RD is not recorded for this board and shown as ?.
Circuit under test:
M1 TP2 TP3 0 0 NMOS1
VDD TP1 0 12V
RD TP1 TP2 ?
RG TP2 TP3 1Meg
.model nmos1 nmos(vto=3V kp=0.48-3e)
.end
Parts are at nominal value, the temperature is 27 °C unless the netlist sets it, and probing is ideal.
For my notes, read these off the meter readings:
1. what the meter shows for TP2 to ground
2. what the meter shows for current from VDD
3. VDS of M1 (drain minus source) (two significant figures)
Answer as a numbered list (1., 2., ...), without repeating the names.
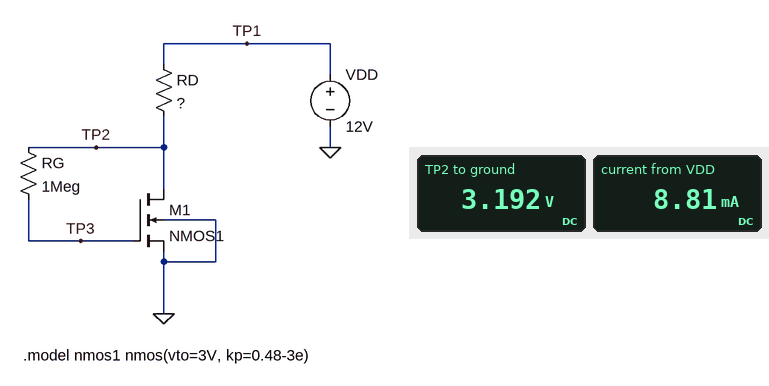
1. 3.192 V
2. 8.81 mA
3. 3.2 V
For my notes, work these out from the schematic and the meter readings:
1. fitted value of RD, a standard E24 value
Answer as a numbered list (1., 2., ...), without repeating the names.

1. 1 kΩ
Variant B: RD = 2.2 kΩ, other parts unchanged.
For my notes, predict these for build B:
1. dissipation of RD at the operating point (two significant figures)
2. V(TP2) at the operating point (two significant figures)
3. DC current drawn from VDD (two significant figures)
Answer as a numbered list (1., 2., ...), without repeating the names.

1. 36 mW
2. 3.1 V
3. 4.0 mA
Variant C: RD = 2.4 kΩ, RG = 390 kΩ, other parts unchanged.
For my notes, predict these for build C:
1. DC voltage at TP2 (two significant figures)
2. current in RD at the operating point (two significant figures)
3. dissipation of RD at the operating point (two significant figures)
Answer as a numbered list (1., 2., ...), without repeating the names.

1. 3.1 V
2. 3.7 mA
3. 33 mW
